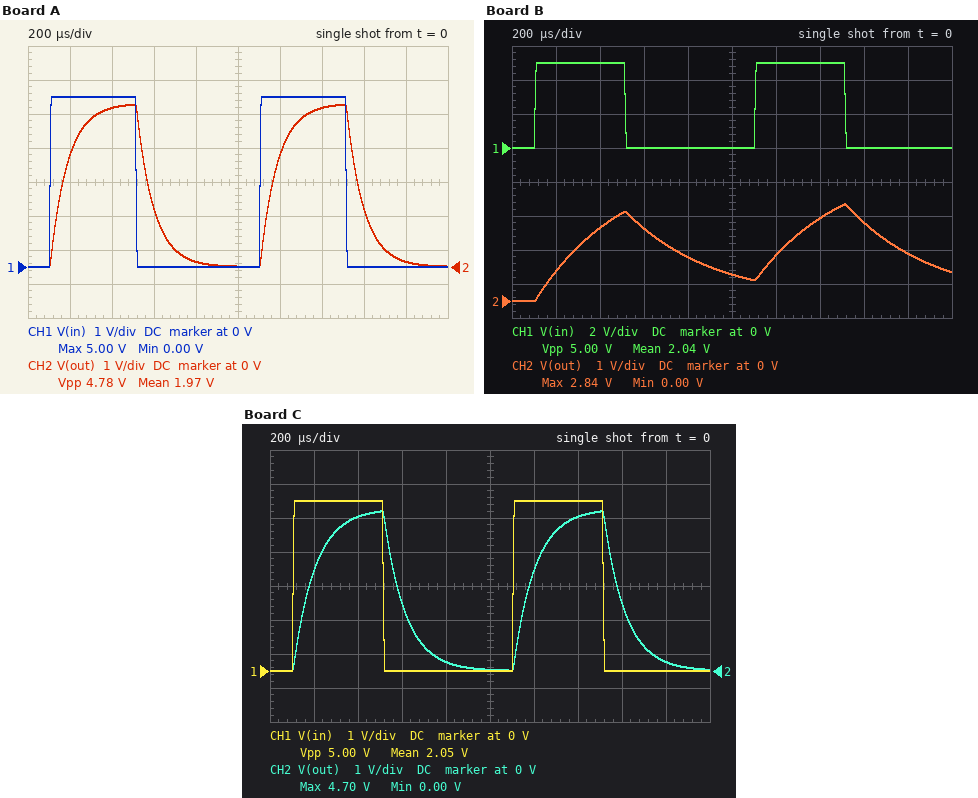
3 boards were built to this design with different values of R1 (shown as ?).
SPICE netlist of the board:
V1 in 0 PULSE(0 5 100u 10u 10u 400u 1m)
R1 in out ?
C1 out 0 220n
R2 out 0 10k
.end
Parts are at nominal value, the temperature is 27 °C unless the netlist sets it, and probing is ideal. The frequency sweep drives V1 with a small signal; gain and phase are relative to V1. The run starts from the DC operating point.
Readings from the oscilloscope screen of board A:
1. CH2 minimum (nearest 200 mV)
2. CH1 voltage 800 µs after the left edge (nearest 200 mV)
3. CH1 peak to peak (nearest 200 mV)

0 V
0 V
5.0 V
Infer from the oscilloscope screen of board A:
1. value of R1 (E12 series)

390 Ω
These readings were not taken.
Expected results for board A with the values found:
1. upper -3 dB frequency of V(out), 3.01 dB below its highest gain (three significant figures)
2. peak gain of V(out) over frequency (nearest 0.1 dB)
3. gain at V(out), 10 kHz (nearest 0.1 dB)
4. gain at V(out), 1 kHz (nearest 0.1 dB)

1.93 kHz
-0.3 dB
-14.8 dB
-1.4 dB
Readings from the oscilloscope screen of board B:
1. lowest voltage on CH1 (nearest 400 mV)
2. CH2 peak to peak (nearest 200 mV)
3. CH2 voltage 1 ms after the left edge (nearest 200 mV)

0 V
2.8 V
800 mV
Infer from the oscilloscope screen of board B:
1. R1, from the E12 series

2.2 kΩ
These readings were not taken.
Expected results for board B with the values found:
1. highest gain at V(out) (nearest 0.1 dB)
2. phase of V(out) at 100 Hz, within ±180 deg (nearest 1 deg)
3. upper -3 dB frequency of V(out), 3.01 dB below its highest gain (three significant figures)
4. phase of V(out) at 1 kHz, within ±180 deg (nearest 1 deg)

-1.7 dB
-14 deg
401 Hz
-68 deg
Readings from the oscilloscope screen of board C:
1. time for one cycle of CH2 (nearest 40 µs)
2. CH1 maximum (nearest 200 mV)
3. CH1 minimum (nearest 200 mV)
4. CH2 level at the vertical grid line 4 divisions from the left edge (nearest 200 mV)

1.00 ms
5.0 V
0 V
200 mV
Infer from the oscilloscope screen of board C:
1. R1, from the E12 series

470 Ω
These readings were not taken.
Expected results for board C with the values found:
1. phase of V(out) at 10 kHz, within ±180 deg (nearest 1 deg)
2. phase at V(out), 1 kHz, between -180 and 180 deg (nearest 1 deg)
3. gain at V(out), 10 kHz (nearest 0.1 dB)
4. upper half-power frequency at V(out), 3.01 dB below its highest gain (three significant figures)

-81 deg
-32 deg
-16.4 dB
1.61 kHz
